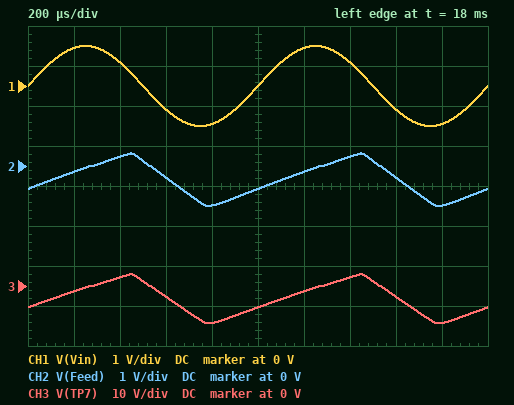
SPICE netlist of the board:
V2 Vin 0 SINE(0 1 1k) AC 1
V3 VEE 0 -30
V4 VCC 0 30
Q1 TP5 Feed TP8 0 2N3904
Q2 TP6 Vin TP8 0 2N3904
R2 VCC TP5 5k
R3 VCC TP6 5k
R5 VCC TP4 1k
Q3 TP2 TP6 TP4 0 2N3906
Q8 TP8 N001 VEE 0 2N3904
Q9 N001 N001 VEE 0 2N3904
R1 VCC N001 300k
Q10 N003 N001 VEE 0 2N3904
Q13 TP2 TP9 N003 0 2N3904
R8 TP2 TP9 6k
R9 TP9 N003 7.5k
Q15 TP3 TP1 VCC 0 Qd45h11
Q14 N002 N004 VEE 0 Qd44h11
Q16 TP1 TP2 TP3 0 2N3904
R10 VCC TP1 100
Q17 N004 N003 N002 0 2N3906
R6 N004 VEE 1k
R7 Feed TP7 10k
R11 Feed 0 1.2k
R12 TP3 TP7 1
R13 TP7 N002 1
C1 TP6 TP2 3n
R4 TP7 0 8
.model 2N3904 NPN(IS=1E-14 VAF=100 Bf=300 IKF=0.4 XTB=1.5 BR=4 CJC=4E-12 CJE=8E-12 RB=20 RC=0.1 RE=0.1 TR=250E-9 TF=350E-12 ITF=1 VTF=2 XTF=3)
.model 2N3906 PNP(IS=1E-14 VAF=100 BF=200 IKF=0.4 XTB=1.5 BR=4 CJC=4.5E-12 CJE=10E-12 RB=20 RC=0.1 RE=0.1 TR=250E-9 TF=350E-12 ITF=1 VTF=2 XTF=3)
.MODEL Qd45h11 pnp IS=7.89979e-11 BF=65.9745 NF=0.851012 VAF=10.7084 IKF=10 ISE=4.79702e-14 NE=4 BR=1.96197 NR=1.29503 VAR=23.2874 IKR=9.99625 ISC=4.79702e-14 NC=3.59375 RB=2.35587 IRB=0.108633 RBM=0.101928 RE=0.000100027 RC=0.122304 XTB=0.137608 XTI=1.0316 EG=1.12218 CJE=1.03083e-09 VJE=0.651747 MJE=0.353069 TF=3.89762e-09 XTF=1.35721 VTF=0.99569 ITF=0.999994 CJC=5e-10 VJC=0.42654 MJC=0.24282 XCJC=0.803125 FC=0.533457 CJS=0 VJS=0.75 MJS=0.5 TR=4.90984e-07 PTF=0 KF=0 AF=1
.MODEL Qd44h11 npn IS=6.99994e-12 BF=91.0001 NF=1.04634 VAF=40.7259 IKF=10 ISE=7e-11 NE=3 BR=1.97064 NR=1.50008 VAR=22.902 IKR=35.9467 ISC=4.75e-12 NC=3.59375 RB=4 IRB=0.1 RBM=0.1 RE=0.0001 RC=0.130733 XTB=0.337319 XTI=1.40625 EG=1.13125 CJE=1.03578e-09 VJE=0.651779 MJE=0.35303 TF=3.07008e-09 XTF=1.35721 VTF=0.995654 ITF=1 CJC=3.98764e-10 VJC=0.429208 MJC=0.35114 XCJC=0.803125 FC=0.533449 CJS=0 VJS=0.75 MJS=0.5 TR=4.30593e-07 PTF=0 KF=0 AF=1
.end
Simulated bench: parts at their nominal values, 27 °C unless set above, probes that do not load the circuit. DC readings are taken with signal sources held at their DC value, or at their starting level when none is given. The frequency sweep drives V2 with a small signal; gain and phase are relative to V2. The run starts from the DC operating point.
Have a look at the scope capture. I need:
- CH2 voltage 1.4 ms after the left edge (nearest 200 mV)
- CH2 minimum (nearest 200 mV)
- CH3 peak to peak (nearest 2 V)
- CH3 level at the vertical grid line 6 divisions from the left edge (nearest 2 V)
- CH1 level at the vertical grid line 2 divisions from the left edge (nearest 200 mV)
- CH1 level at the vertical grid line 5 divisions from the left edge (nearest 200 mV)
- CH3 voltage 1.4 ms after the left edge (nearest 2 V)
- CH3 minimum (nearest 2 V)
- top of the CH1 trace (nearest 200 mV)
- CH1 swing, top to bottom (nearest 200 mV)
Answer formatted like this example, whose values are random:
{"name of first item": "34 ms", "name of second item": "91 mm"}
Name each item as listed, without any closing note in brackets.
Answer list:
{"CH2 voltage 1.4 ms after the left edge": "200 mV", "CH2 minimum": "-1.0 V", "CH3 peak to peak": "12 V", "CH3 level at the vertical grid line 6 divisions from the left edge": "-2 V", "CH1 level at the vertical grid line 2 divisions from the left edge": "600 mV", "CH1 level at the vertical grid line 5 divisions from the left edge": "0 V", "CH3 voltage 1.4 ms after the left edge": "2 V", "CH3 minimum": "-10 V", "top of the CH1 trace": "1.0 V", "CH1 swing, top to bottom": "2.0 V"}
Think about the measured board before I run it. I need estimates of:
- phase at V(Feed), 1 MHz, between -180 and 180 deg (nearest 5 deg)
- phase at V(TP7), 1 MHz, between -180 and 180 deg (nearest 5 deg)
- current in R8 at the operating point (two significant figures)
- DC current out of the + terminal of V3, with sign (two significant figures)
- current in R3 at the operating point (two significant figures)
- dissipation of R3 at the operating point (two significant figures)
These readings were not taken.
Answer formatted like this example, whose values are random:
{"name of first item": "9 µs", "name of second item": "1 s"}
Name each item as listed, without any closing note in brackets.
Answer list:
{"phase at V(Feed), 1 MHz, between -180 and 180 deg": "120 deg", "phase at V(TP7), 1 MHz, between -180 and 180 deg": "160 deg", "current in R8 at the operating point": "82 µA", "DC current out of the + terminal of V3, with sign": "-25 mA", "current in R3 at the operating point": "170 µA", "dissipation of R3 at the operating point": "150 µW"}
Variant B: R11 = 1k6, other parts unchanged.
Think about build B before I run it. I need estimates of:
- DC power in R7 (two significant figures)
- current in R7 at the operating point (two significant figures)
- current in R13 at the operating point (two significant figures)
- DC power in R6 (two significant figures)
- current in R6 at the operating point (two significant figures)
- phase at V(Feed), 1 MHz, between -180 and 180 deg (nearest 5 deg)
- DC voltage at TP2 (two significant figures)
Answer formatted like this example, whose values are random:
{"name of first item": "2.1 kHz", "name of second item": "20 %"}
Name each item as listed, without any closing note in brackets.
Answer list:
{"DC power in R7": "1.6 µW", "current in R7 at the operating point": "13 µA", "current in R13 at the operating point": "19 mA", "DC power in R6": "330 µW", "current in R6 at the operating point": "570 µA", "phase at V(Feed), 1 MHz, between -180 and 180 deg": "115 deg", "DC voltage at TP2": "290 mV"}
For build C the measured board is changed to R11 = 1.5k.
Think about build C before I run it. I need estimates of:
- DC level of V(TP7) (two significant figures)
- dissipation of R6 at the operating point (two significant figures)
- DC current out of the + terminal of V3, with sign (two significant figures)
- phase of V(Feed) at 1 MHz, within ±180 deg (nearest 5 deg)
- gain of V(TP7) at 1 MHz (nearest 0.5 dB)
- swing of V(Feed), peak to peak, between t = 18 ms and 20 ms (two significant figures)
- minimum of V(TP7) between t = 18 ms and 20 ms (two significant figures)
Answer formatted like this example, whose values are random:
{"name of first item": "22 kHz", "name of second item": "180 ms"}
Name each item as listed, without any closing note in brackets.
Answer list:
{"DC level of V(TP7)": "-160 mV", "dissipation of R6 at the operating point": "330 µW", "DC current out of the + terminal of V3, with sign": "-20 mA", "phase of V(Feed) at 1 MHz, within ±180 deg": "115 deg", "gain of V(TP7) at 1 MHz": "6.0 dB", "swing of V(Feed), peak to peak, between t = 18 ms and 20 ms": "1.5 V", "minimum of V(TP7) between t = 18 ms and 20 ms": "-7.8 V"}
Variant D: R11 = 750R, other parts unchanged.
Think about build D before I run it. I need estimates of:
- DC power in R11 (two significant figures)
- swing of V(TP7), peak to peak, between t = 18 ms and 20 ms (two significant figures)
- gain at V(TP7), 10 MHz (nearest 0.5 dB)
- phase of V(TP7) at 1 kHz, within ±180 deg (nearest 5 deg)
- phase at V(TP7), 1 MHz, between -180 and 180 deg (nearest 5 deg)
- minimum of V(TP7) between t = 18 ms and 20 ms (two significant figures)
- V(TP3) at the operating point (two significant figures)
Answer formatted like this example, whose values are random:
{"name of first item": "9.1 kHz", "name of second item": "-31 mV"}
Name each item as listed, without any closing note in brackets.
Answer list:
{"DC power in R11": "570 nW", "swing of V(TP7), peak to peak, between t = 18 ms and 20 ms": "13 V", "gain at V(TP7), 10 MHz": "-10.5 dB", "phase of V(TP7) at 1 kHz, within ±180 deg": "-10 deg", "phase at V(TP7), 1 MHz, between -180 and 180 deg": "165 deg", "minimum of V(TP7) between t = 18 ms and 20 ms": "-12 V", "V(TP3) at the operating point": "-290 mV"}
